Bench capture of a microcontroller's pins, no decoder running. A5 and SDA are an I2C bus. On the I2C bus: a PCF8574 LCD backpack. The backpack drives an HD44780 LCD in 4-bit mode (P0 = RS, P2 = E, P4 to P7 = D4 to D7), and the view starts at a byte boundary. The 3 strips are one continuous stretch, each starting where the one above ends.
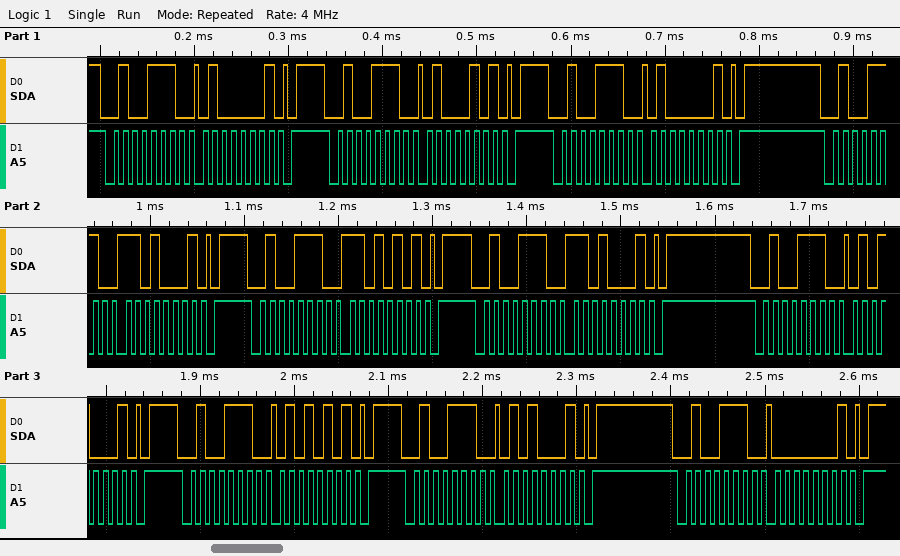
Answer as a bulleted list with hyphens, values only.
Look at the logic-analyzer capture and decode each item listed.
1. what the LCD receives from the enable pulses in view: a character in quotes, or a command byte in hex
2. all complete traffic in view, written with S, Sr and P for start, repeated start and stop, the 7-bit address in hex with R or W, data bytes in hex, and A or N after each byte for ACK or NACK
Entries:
- 'M'
- S 27W A 41 A P S 27W A 45 A P S 27W A 41 A P S 27W A D1 A P S 27W A D5 A P S 27W A D1 A P S 27W A 51 A P S 27W A 55 A P S 27W A 51 A P S 27W A 01 A P
